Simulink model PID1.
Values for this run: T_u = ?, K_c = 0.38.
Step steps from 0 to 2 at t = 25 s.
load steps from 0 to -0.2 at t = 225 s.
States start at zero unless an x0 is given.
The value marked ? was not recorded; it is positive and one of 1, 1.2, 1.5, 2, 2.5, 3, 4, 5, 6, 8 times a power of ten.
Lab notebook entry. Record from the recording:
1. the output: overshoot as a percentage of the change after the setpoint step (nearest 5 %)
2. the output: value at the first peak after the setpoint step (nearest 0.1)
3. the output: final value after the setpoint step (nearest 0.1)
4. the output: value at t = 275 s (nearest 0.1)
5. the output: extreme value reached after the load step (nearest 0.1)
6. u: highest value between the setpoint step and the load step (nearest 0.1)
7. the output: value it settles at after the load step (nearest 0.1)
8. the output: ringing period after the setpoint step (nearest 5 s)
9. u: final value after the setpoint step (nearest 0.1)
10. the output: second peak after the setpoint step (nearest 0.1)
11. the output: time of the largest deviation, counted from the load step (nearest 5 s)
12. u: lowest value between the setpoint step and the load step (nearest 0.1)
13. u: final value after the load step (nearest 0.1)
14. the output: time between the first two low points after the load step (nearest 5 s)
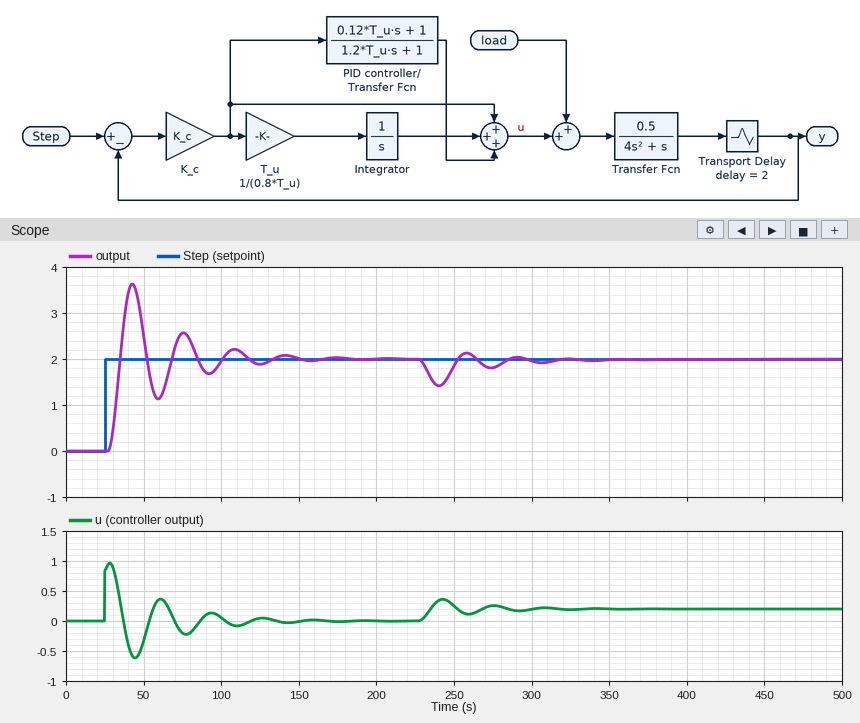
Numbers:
80 %
3.6
2.0
1.8
1.4
1.0
2.0
35 s
0.0
2.6
15 s
-0.6
0.2
35 s
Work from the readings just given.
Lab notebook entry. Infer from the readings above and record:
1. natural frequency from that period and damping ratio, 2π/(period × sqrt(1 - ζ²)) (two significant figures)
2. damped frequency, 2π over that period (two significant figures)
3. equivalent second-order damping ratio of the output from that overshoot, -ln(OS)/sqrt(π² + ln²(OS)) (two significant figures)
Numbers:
0.18 rad/s
0.18 rad/s
0.071
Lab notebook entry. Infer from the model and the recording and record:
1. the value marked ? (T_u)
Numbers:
30
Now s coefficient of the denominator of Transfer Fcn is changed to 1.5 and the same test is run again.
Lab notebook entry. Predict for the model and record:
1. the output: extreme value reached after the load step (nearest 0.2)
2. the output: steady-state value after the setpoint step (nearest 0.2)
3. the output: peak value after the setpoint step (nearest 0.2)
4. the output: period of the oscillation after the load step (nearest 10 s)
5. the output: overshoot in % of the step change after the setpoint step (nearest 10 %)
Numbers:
1.6
2.0
3.0
40 s
50 %
